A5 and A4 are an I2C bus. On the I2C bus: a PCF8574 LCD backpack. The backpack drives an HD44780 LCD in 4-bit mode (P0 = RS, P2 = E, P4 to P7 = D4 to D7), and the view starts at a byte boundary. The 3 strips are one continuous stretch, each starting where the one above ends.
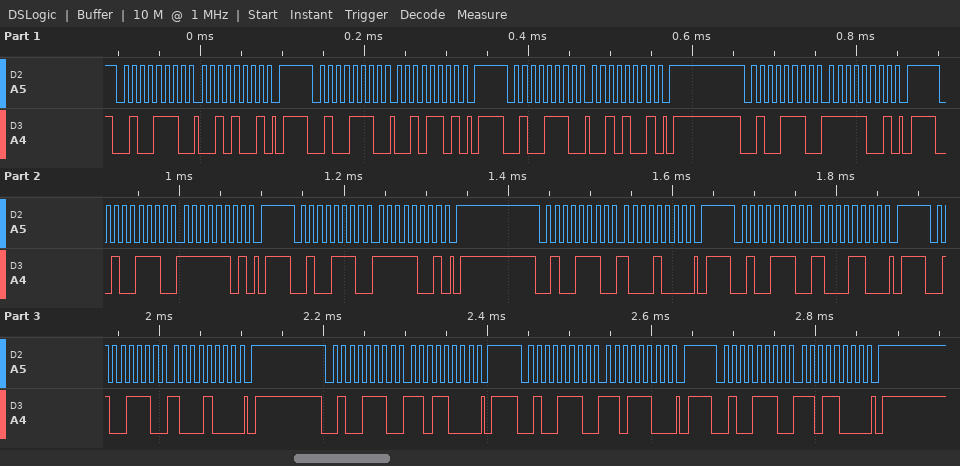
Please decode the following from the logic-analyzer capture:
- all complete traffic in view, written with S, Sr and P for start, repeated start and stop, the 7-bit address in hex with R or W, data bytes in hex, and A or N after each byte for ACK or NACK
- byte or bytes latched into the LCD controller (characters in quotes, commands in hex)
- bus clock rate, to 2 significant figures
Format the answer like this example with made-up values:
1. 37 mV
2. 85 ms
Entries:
1. S 27W A 29 A P S 27W A 2D A P S 27W A 29 A P S 27W A F9 A P S 27W A FD A P S 27W A F9 A P S 27W A 88 A P S 27W A 8C A P S 27W A 88 A P S 27W A D8 A P S 27W A DC A P S 27W A D8 A P
2. '/' 0x8D
3. 100 kHz
